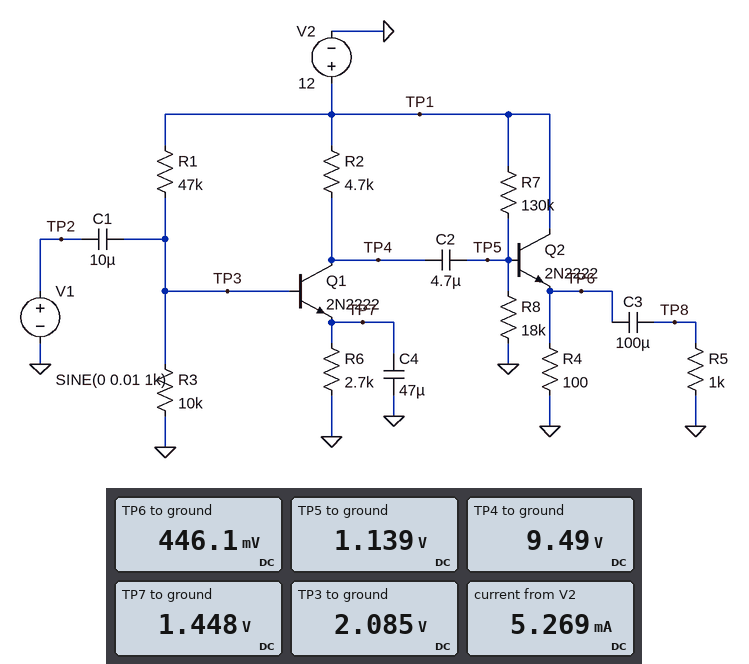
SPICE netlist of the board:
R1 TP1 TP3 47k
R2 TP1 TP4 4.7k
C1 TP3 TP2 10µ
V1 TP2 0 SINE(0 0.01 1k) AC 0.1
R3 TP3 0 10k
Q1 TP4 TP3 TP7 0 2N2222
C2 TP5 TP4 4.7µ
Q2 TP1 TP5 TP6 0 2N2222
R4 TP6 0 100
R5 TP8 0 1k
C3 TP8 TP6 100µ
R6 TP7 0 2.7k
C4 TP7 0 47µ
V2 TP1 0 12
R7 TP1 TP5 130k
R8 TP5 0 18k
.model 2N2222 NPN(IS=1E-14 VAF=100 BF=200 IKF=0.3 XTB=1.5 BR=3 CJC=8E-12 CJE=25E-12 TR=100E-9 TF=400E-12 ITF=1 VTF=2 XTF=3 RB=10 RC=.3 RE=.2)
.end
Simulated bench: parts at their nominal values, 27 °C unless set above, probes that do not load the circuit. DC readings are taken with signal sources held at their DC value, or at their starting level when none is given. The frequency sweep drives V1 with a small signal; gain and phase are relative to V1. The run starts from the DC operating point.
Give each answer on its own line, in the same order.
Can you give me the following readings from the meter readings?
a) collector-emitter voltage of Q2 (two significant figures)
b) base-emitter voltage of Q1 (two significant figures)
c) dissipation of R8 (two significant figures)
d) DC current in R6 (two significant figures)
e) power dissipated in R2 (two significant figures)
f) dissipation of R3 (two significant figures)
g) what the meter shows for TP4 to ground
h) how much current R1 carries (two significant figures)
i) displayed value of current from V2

12 V
640 mV
72 µW
540 µA
1.3 mW
430 µW
9.49 V
210 µA
5.269 mA
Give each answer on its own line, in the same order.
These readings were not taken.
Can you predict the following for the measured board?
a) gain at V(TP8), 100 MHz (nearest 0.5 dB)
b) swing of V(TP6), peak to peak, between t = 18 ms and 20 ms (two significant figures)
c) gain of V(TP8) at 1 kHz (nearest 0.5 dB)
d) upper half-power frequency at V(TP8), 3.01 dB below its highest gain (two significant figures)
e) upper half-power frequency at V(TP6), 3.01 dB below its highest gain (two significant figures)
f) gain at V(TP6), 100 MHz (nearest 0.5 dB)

6.5 dB
930 mV
35.5 dB
3.7 MHz
3.7 MHz
6.5 dB
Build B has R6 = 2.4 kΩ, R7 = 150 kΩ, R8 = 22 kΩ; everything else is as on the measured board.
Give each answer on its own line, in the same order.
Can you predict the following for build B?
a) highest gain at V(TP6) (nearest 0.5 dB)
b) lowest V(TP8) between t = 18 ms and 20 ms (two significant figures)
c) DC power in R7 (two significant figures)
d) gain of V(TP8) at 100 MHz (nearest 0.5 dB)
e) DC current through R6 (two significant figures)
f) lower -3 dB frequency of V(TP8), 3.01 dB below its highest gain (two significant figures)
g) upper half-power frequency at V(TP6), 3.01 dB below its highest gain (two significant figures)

36.5 dB
-420 mV
790 µW
7.5 dB
600 µA
80 Hz
3.5 MHz
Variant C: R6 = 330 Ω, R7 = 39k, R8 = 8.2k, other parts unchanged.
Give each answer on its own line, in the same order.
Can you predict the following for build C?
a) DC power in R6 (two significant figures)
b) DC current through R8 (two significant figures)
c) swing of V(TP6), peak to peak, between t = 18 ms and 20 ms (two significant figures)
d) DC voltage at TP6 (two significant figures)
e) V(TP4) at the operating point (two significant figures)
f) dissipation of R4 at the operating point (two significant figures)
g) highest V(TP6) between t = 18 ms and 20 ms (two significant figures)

2.0 mW
210 µA
1.5 V
1.0 V
880 mV
11 mW
2.3 V
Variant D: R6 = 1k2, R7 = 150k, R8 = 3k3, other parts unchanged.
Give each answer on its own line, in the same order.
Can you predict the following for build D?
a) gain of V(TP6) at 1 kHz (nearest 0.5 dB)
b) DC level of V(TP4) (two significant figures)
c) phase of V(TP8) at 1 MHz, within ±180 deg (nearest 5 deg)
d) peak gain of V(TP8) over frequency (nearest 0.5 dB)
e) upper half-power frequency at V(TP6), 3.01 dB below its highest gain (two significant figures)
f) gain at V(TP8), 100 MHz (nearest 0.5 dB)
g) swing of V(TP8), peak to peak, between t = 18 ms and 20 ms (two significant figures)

-57.5 dB
6.5 V
-115 deg
9.5 dB
160 MHz
8.0 dB
290 mV
